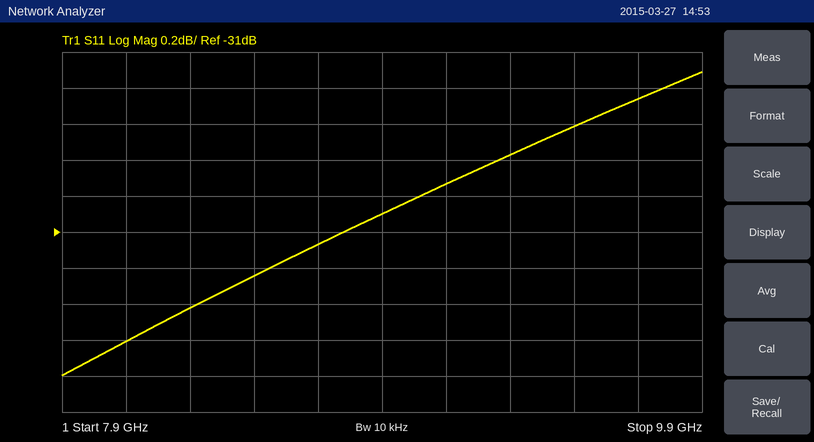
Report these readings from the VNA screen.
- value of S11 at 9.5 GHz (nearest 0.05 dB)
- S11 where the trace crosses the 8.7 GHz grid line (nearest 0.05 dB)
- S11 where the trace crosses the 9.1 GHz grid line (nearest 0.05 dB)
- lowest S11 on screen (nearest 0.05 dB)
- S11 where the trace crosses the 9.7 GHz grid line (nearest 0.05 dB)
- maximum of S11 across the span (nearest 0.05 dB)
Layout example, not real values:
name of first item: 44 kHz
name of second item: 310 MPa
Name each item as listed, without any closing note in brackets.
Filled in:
value of S11 at 9.5 GHz: -30.40 dB
S11 where the trace crosses the 8.7 GHz grid line: -31.05 dB
S11 where the trace crosses the 9.1 GHz grid line: -30.75 dB
lowest S11 on screen: -31.80 dB
S11 where the trace crosses the 9.7 GHz grid line: -30.25 dB
maximum of S11 across the span: -30.10 dB
